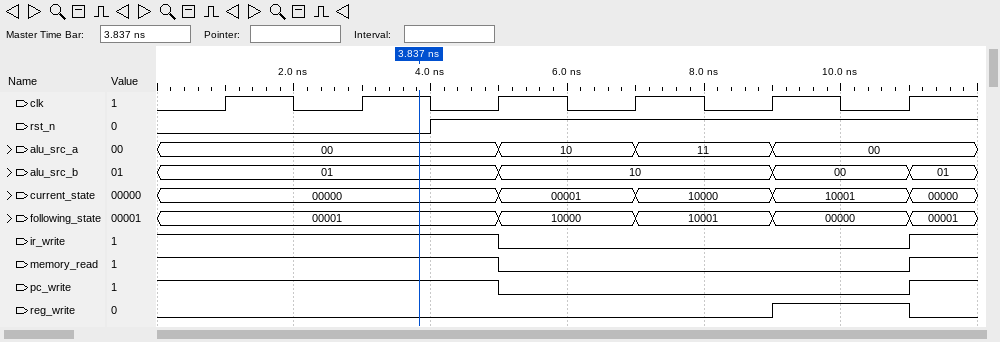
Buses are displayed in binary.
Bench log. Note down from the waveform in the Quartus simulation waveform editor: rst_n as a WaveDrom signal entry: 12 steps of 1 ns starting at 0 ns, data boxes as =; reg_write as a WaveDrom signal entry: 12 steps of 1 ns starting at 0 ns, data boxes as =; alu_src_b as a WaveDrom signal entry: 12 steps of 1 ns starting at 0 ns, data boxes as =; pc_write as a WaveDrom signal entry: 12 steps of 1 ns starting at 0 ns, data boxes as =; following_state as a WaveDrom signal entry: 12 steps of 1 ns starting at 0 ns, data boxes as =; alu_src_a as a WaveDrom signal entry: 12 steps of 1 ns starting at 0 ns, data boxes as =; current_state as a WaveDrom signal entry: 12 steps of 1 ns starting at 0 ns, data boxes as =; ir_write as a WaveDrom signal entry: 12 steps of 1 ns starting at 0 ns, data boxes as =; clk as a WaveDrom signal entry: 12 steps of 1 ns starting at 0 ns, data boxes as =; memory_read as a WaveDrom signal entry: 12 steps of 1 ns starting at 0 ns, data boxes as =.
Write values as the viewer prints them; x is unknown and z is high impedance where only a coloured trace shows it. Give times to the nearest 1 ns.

{name: 'rst_n', wave: '0...1.......'}
{name: 'reg_write', wave: '0........1.0'}
{name: 'alu_src_b', wave: '=....=...=.=', data: '01 10 00 01'}
{name: 'pc_write', wave: '1....0.....1'}
{name: 'following_state', wave: '=....=.=.=.=', data: '00001 10000 10001 00000 00001'}
{name: 'alu_src_a', wave: '=....=.=.=..', data: '00 10 11 00'}
{name: 'current_state', wave: '=....=.=.=.=', data: '00000 00001 10000 10001 00000'}
{name: 'ir_write', wave: '1....0.....1'}
{name: 'clk', wave: '010101010101'}
{name: 'memory_read', wave: '1....0.....1'}
